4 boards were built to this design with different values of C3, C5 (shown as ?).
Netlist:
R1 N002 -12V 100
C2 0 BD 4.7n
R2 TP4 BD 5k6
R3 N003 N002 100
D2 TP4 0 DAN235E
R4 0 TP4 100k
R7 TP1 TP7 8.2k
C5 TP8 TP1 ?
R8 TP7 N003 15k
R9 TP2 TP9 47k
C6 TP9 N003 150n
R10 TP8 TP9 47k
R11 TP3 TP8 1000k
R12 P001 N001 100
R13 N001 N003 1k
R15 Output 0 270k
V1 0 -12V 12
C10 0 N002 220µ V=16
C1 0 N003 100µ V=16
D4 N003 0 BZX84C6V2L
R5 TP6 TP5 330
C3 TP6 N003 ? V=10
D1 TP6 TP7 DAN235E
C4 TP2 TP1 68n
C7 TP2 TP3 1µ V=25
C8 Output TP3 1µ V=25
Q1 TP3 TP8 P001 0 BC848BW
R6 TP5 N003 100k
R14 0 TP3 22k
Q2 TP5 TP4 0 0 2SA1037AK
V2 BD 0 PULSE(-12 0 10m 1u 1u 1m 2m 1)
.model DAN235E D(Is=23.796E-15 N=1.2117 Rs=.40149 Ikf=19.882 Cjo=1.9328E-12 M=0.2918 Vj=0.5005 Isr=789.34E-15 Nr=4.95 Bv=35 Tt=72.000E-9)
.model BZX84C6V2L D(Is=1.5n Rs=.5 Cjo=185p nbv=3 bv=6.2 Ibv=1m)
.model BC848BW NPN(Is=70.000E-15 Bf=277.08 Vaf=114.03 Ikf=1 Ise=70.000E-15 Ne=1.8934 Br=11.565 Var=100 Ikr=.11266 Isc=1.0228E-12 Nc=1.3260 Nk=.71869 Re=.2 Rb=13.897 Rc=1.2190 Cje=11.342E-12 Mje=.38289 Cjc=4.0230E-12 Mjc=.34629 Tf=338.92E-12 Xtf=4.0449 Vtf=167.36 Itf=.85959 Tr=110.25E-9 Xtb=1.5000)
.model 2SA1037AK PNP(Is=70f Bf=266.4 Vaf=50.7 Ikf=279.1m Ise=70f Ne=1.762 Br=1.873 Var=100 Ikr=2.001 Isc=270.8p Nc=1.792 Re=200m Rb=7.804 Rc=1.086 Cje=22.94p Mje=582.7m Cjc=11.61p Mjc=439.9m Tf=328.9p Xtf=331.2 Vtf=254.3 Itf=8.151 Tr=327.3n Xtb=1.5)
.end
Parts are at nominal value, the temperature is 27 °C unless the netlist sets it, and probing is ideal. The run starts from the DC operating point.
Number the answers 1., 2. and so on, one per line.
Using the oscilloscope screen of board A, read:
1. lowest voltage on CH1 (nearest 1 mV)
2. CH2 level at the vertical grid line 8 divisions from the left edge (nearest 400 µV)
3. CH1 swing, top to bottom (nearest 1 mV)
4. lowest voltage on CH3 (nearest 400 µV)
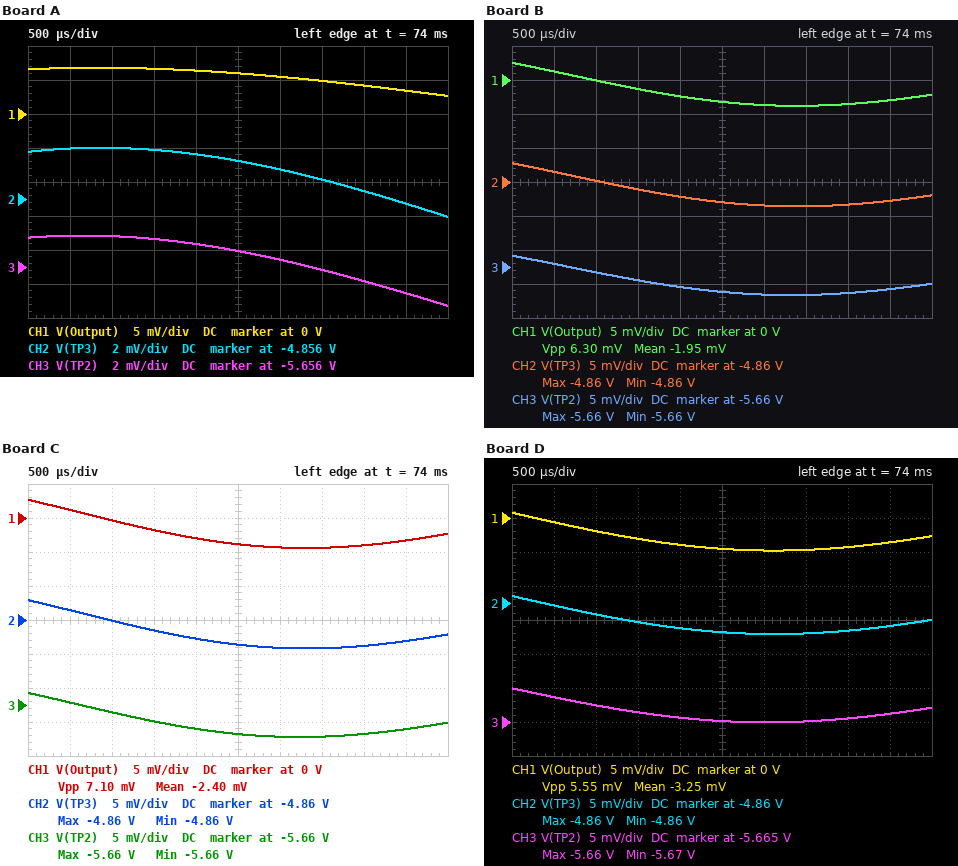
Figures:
1. 3 mV
2. -4.8556 V
3. 4 mV
4. -5.6584 V
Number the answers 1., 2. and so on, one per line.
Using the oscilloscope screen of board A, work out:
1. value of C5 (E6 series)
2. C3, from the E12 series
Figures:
1. 150 nF
2. 6.8 µF
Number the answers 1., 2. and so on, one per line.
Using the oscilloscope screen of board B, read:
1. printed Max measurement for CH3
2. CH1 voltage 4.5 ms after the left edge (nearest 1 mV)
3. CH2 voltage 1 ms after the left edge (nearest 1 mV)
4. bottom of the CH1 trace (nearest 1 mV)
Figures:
1. -5.66 V
2. -3 mV
3. -4.860 V
4. -4 mV
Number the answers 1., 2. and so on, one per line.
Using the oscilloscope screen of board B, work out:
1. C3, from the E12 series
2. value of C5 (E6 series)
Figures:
1. 8.2 µF
2. 22 nF
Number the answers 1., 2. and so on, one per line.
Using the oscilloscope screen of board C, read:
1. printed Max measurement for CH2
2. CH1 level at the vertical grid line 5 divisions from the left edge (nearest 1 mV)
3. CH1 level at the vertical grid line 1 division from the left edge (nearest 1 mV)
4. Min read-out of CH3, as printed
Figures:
1. -4.86 V
2. -4 mV
3. 1 mV
4. -5.66 V
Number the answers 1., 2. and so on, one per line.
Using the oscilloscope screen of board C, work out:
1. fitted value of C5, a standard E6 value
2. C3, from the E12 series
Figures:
1. 22 nF
2. 6.8 µF
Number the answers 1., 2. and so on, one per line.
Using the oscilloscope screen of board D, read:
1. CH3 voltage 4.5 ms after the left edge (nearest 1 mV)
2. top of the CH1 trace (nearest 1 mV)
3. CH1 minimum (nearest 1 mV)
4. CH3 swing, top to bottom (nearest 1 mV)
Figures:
1. -5.664 V
2. 1 mV
3. -5 mV
4. 5 mV
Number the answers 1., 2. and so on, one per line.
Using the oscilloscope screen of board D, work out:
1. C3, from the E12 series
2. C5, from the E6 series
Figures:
1. 22 µF
2. 33 nF
